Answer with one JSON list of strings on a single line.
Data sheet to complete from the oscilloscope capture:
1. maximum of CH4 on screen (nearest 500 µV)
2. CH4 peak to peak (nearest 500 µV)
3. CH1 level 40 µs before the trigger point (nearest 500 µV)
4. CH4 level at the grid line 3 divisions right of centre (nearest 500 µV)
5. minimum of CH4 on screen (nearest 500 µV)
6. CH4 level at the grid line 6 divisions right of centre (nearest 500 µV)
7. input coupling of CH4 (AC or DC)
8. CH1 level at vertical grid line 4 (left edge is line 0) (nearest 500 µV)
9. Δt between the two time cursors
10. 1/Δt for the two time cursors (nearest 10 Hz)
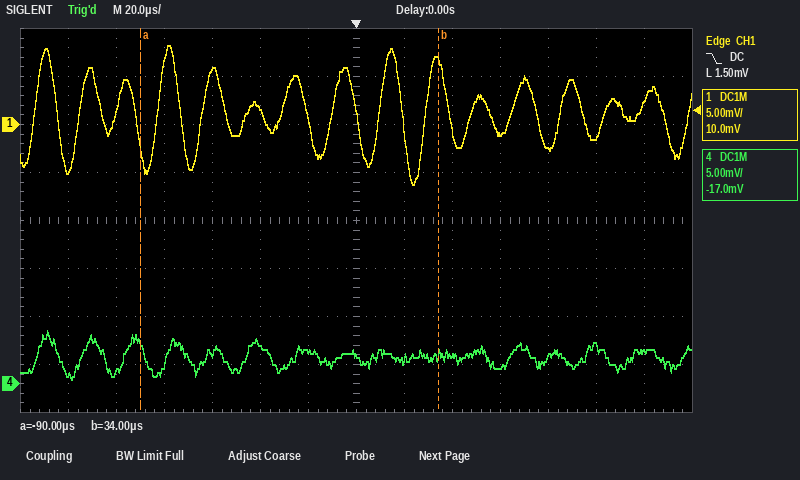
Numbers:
["5.5 mV", "5.0 mV", "1.5 mV", "1.5 mV", "500 µV", "3.5 mV", "DC", "5.5 mV", "124 µs", "8.06 kHz"]
